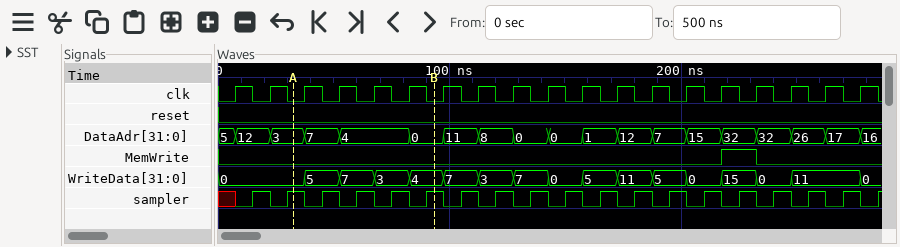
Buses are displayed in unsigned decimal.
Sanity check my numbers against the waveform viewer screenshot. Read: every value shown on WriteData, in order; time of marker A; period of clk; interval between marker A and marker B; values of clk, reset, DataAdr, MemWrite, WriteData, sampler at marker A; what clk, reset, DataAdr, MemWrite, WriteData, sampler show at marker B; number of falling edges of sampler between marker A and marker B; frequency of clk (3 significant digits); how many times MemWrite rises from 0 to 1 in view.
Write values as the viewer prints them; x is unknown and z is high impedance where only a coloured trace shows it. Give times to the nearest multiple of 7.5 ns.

0, 5, 7, 3, 4, 7, 3, 7, 0, 5, 11, 5, 0, 15, 0, 11, 0
30 ns
15 ns
60 ns
clk=0, reset=0, DataAdr=3, MemWrite=0, WriteData=0, sampler=1
clk=0, reset=0, DataAdr=0, MemWrite=0, WriteData=4, sampler=1
4
66.7 MHz
1
